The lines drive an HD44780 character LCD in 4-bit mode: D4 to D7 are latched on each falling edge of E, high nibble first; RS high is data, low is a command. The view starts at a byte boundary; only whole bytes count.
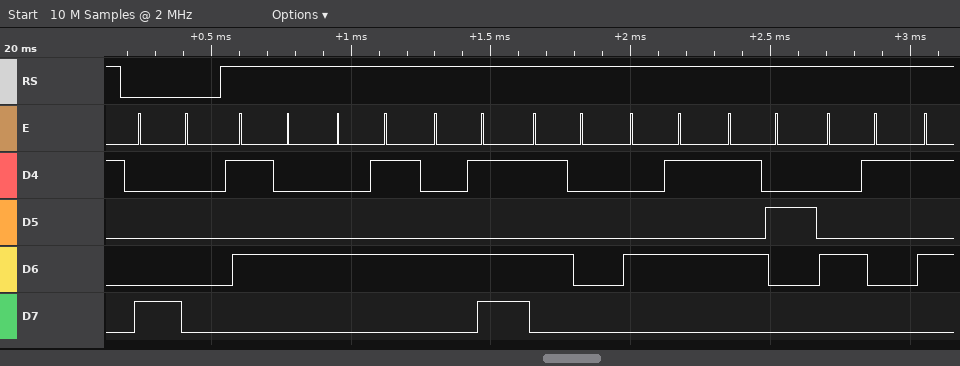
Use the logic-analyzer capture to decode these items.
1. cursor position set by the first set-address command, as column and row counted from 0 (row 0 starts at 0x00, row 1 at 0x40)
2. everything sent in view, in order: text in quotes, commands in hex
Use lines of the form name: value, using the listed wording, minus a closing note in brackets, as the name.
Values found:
cursor position set by the first set-address command, as column and row counted from 0: column 0, row 0
everything sent in view, in order: text in quotes, commands in hex: 0x80 "TEMPERA"
